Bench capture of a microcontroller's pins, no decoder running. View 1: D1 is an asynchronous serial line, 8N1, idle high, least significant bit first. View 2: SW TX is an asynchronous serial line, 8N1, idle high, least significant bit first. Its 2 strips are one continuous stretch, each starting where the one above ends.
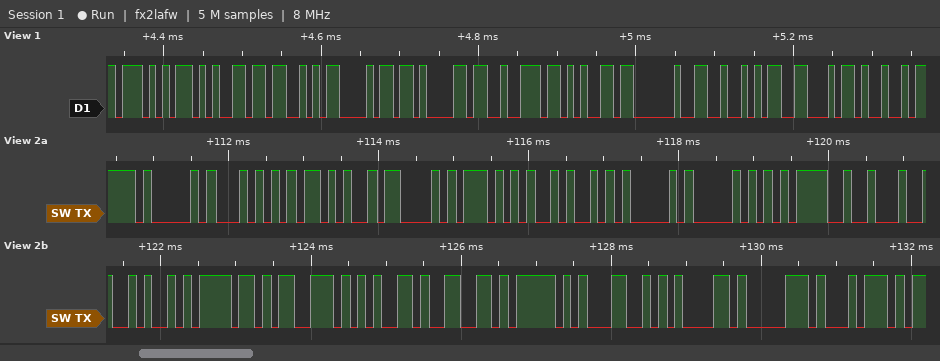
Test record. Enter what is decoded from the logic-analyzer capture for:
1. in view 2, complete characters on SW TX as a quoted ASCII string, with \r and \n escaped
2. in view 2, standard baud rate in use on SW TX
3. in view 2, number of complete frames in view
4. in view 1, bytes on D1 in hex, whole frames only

"AT+CWJAP=\"Josef_Lapt"
9600 baud
20
0x57 0x65 0x53 0x68 0x61 0x72 0x65 0x20 0x52 0x46 0x49
